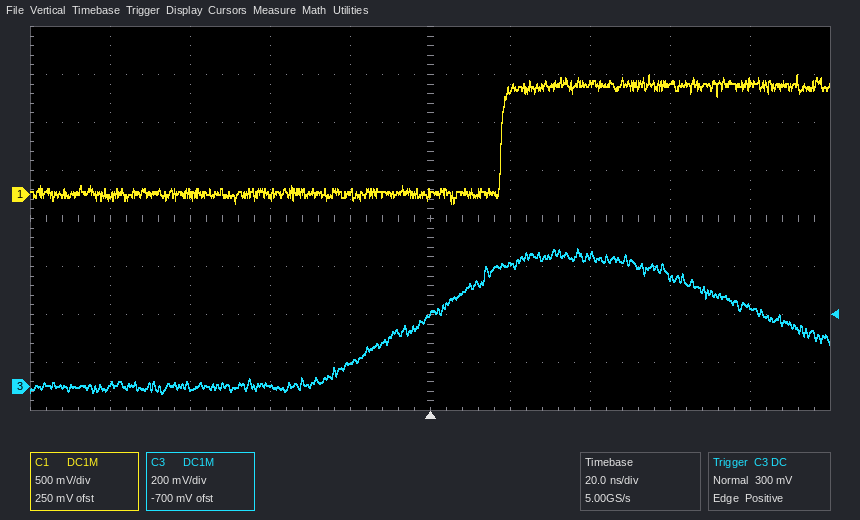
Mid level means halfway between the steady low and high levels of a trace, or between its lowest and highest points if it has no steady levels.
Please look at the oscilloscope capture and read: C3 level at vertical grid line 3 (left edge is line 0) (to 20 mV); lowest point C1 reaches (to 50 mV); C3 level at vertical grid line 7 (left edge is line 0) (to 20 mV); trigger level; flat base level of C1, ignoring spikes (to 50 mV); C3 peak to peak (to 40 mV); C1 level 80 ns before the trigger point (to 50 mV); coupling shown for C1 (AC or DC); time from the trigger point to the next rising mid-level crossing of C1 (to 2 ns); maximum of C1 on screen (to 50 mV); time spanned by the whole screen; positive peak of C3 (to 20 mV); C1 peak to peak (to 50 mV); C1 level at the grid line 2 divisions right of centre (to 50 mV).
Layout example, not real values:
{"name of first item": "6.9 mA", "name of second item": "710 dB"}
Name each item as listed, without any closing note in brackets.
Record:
{"C3 level at vertical grid line 3 (left edge is line 0)": "0 mV", "lowest point C1 reaches": "-100 mV", "C3 level at vertical grid line 7 (left edge is line 0)": "540 mV", "trigger level": "300 mV", "flat base level of C1, ignoring spikes": "0 mV", "C3 peak to peak": "600 mV", "C1 level 80 ns before the trigger point": "0 mV", "coupling shown for C1": "DC", "time from the trigger point to the next rising mid-level crossing of C1": "18 ns", "maximum of C1 on screen": "1.25 V", "time spanned by the whole screen": "200 ns", "positive peak of C3": "580 mV", "C1 peak to peak": "1.35 V", "C1 level at the grid line 2 divisions right of centre": "1.15 V"}
